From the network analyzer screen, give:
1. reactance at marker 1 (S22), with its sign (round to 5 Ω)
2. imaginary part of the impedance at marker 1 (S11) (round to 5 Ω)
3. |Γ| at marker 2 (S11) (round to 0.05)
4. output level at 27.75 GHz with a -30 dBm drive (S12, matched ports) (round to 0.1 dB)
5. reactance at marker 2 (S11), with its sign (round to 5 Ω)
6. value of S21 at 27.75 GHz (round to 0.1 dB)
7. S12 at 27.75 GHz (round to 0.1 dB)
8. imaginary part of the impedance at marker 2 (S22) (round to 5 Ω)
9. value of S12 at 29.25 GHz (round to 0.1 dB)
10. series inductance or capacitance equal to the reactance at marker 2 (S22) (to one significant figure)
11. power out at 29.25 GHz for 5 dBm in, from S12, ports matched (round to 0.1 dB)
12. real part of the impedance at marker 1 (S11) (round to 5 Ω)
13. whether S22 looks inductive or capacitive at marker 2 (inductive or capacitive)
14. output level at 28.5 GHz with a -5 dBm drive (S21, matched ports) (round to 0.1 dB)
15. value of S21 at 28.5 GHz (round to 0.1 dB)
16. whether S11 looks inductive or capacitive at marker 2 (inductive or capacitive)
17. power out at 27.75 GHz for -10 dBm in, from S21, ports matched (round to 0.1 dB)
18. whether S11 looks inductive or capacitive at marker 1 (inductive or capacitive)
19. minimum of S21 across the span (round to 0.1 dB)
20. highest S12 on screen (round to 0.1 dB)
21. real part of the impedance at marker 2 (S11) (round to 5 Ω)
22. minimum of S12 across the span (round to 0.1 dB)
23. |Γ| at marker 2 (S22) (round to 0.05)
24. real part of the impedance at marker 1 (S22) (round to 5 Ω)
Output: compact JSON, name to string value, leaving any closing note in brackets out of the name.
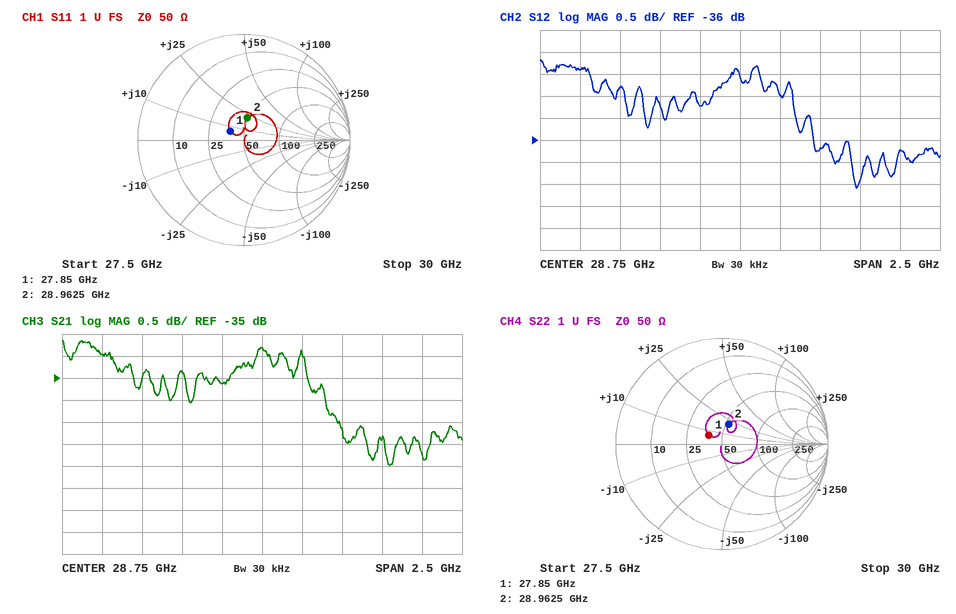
{"reactance at marker 1 (S22), with its sign": "+5 Ω", "imaginary part of the impedance at marker 1 (S11)": "+5 Ω", "|Γ| at marker 2 (S11)": "0.20", "output level at 27.75 GHz with a -30 dBm drive (S12, matched ports)": "-64.4 dBm", "reactance at marker 2 (S11), with its sign": "+20 Ω", "value of S21 at 27.75 GHz": "-34.5 dB", "S12 at 27.75 GHz": "-34.4 dB", "imaginary part of the impedance at marker 2 (S22)": "+20 Ω", "value of S12 at 29.25 GHz": "-36.2 dB", "series inductance or capacitance equal to the reactance at marker 2 (S22)": "100 pH", "power out at 29.25 GHz for 5 dBm in, from S12, ports matched": "-31.2 dBm", "real part of the impedance at marker 1 (S11)": "40 Ω", "whether S22 looks inductive or capacitive at marker 2": "inductive", "output level at 28.5 GHz with a -5 dBm drive (S21, matched ports)": "-40.1 dBm", "value of S21 at 28.5 GHz": "-35.1 dB", "whether S11 looks inductive or capacitive at marker 2": "inductive", "power out at 27.75 GHz for -10 dBm in, from S21, ports matched": "-44.5 dBm", "whether S11 looks inductive or capacitive at marker 1": "inductive", "minimum of S21 across the span": "-37.0 dB", "highest S12 on screen": "-34.2 dB", "real part of the impedance at marker 2 (S11)": "50 Ω", "minimum of S12 across the span": "-37.1 dB", "|Γ| at marker 2 (S22)": "0.20", "real part of the impedance at marker 1 (S22)": "40 Ω"}
